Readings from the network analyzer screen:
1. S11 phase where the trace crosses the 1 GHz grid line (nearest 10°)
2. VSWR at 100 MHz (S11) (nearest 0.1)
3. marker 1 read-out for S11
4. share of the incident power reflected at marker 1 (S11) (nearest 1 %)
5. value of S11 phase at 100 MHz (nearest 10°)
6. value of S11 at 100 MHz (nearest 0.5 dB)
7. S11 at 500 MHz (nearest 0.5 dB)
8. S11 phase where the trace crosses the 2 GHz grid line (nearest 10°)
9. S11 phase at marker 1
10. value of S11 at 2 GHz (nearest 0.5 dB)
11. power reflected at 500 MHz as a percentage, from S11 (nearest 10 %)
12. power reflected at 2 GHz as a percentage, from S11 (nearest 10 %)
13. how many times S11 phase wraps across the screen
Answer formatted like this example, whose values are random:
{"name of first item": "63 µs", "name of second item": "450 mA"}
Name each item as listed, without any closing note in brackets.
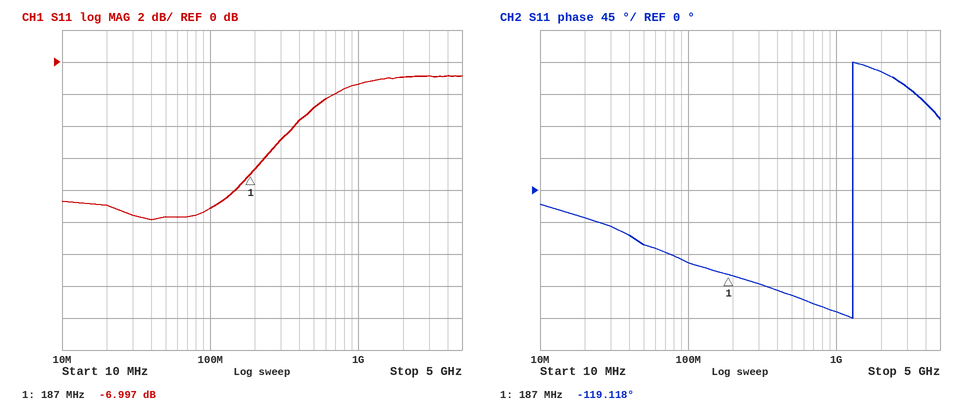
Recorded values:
{"S11 phase where the trace crosses the 1 GHz grid line": "-170°", "VSWR at 100 MHz (S11)": "2.1", "marker 1 read-out for S11": "-6.997 dB", "share of the incident power reflected at marker 1 (S11)": "20 %", "value of S11 phase at 100 MHz": "-100°", "value of S11 at 100 MHz": "-9.0 dB", "S11 at 500 MHz": "-3.0 dB", "S11 phase where the trace crosses the 2 GHz grid line": "170°", "S11 phase at marker 1": "-119.118°", "value of S11 at 2 GHz": "-1.0 dB", "power reflected at 500 MHz as a percentage, from S11": "50 %", "power reflected at 2 GHz as a percentage, from S11": "80 %", "how many times S11 phase wraps across the screen": "1"}
